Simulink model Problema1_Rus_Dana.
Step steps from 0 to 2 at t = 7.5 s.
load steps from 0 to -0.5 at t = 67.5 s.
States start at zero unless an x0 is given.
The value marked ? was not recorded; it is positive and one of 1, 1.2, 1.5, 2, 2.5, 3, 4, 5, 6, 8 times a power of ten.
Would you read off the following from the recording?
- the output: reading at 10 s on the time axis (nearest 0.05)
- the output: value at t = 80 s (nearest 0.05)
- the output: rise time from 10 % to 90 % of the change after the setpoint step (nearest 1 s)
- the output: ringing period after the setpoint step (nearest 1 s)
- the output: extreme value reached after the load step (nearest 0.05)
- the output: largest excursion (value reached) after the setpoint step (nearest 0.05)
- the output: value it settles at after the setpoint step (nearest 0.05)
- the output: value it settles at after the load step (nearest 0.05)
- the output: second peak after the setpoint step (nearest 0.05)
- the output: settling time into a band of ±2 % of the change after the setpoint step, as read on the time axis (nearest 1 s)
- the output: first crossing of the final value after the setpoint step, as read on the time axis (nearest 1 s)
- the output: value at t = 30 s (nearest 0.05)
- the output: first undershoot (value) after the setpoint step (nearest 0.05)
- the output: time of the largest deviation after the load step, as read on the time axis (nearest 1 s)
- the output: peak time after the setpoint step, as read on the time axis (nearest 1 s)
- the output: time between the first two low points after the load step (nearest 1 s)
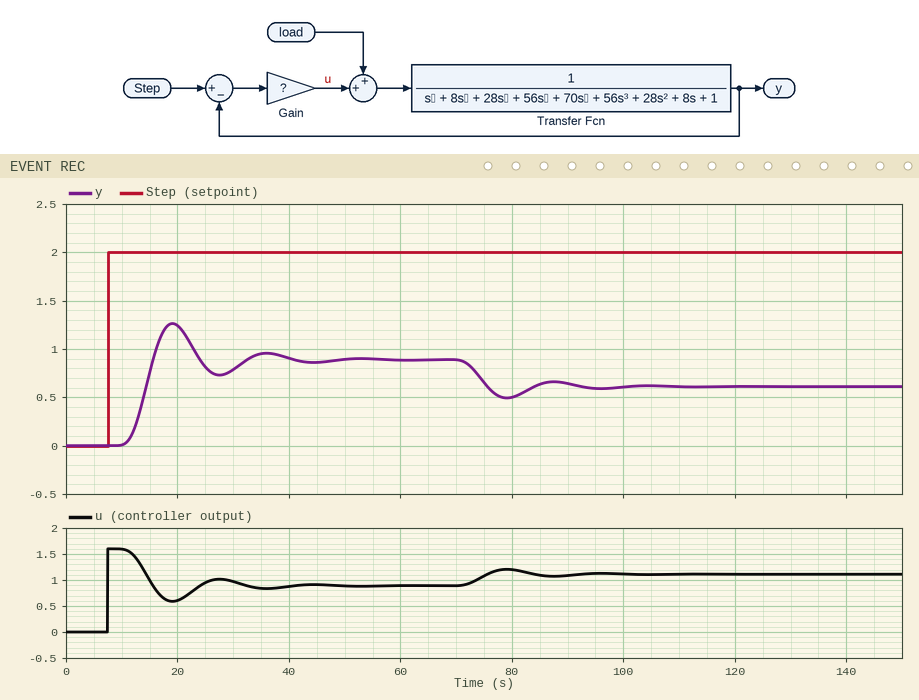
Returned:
0.00
0.50
4 s
17 s
0.50
1.25
0.90
0.60
0.95
47 s
16 s
0.80
0.75
79 s
19 s
17 s
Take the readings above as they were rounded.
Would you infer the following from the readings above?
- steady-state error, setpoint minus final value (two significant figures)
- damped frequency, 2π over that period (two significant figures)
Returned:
1.1
0.37 rad/s
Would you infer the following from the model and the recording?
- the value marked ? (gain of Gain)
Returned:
0.8
